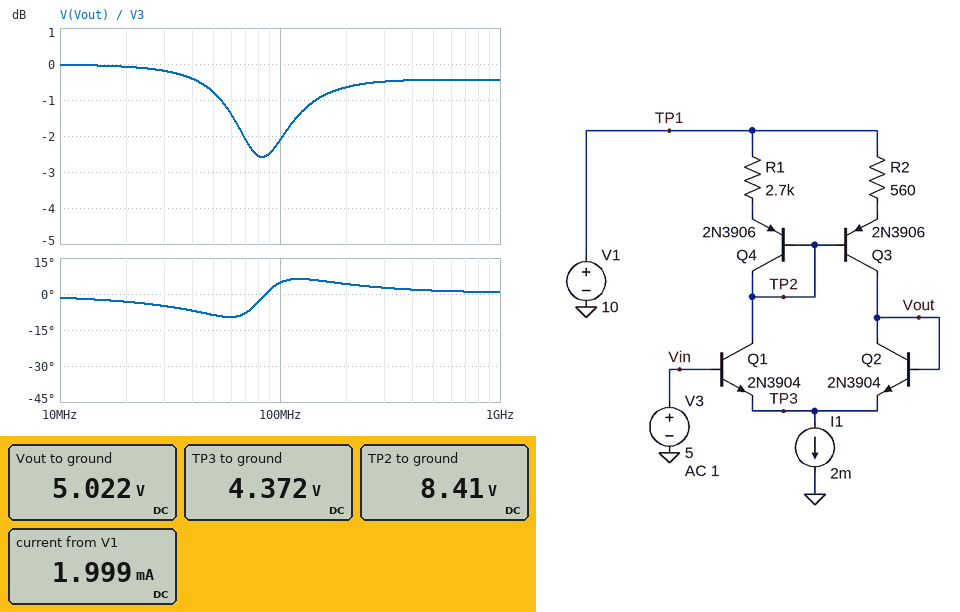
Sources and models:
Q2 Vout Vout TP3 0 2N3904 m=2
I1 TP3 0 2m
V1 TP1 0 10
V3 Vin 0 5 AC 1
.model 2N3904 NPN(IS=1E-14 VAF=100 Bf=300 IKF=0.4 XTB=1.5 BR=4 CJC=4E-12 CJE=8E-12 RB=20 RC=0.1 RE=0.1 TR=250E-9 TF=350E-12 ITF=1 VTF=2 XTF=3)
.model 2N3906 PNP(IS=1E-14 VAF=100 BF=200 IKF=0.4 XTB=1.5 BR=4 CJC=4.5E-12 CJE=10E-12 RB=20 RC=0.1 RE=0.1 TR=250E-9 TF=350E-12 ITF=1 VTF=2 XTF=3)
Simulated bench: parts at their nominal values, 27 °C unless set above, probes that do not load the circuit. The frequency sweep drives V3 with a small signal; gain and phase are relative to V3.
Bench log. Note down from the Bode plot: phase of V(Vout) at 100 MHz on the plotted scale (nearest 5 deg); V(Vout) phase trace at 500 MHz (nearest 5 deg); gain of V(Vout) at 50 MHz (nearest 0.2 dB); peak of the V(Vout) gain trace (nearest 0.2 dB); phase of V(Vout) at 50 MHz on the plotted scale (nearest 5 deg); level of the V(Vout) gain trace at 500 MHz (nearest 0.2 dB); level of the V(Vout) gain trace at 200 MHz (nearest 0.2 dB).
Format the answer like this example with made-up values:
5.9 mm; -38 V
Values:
5 deg; 0 deg; -0.8 dB; 0 dB; -10 deg; -0.4 dB; -0.6 dB
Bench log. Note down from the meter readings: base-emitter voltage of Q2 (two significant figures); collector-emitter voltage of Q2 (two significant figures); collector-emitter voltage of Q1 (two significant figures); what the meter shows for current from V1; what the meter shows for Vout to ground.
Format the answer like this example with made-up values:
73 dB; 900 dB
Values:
650 mV; 650 mV; 4.0 V; 1.999 mA; 5.022 V
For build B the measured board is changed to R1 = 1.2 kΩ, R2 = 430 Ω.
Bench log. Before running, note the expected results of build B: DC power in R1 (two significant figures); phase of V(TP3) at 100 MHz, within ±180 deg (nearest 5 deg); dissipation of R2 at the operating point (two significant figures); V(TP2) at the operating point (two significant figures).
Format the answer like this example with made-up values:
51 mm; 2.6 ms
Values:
350 µW; -5 deg; 910 µW; 8.7 V
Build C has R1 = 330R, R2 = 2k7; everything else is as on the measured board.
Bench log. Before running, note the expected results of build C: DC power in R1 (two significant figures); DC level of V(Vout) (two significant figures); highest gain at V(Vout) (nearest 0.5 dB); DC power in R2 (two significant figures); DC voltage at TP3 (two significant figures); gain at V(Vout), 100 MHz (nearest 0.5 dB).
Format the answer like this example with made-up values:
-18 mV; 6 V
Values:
1.0 mW; 4.9 V; 0 dB; 150 µW; 4.3 V; -1.0 dB
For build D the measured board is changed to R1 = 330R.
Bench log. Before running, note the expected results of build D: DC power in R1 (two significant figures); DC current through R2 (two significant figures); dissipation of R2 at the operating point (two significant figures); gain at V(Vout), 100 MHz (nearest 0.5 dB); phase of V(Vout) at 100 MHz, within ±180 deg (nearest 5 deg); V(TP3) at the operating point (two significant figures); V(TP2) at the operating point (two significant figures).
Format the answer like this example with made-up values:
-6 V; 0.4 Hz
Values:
510 µW; 760 µA; 320 µW; -1.0 dB; -5 deg; 4.3 V; 8.9 V
